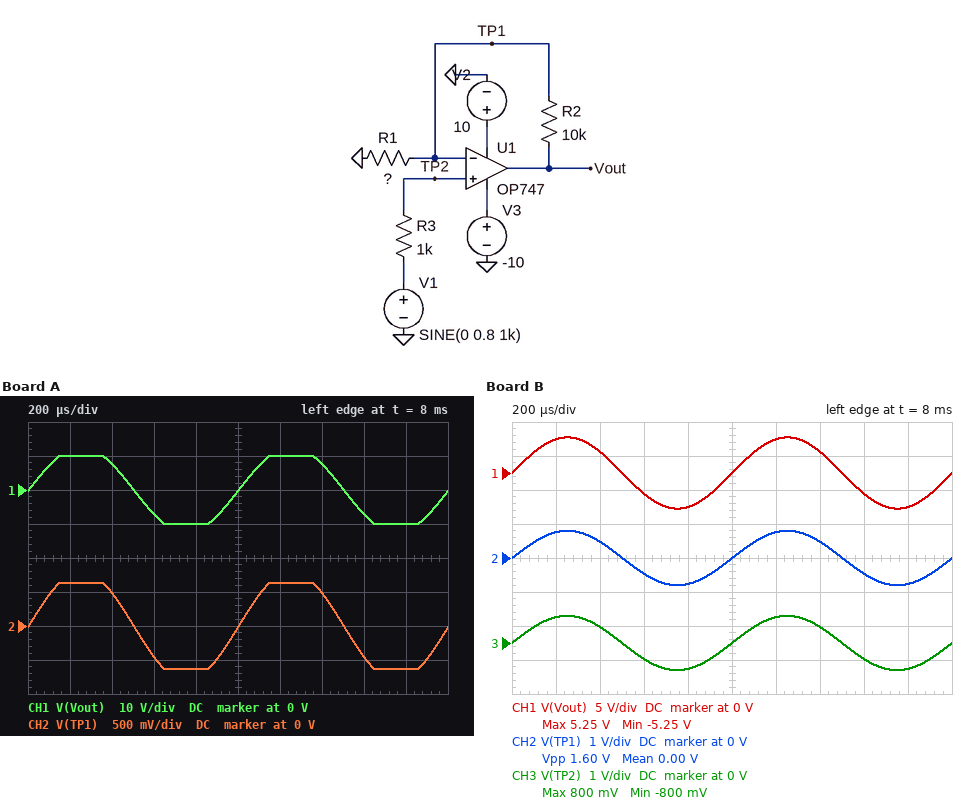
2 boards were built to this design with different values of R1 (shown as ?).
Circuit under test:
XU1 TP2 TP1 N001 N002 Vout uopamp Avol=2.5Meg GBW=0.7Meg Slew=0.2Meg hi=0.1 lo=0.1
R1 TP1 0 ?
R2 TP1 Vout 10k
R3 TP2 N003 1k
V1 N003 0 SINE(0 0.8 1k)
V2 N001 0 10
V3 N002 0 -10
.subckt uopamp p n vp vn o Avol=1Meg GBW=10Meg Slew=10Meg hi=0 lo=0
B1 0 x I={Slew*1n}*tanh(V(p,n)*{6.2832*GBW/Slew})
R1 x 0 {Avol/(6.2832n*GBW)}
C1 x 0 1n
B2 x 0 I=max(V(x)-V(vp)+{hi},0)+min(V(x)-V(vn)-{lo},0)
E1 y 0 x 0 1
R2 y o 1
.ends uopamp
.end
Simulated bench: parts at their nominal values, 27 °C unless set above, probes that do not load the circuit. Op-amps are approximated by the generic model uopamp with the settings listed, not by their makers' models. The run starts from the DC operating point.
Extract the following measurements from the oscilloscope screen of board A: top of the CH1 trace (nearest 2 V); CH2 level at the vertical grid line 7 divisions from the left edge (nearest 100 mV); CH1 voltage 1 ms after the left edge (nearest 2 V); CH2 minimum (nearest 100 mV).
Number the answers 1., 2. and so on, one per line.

1. 10 V
2. 500 mV
3. 0 V
4. -600 mV
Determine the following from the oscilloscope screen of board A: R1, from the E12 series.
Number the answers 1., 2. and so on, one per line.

1. 680 Ω
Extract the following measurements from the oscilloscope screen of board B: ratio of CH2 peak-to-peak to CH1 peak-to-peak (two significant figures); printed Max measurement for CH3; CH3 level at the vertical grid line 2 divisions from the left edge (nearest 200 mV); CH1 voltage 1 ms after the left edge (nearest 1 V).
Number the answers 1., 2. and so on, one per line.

1. 0.15
2. 800 mV
3. 400 mV
4. 0 V
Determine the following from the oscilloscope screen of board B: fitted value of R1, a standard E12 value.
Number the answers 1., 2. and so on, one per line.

1. 1.8 kΩ
